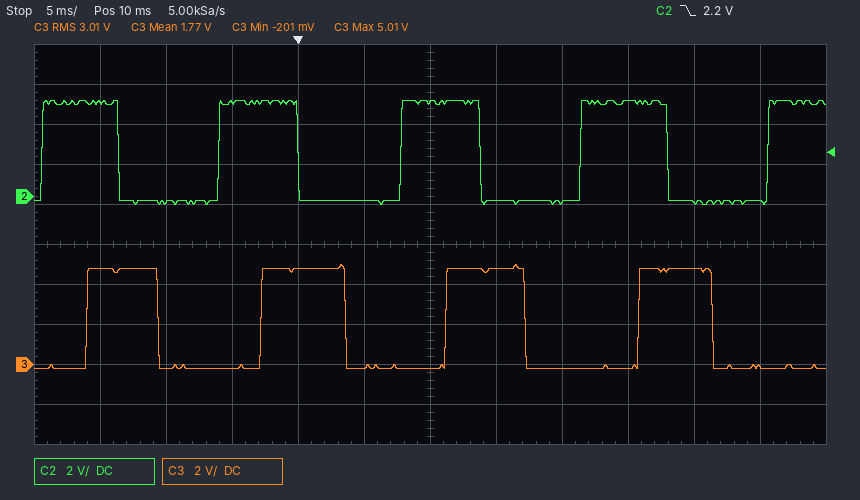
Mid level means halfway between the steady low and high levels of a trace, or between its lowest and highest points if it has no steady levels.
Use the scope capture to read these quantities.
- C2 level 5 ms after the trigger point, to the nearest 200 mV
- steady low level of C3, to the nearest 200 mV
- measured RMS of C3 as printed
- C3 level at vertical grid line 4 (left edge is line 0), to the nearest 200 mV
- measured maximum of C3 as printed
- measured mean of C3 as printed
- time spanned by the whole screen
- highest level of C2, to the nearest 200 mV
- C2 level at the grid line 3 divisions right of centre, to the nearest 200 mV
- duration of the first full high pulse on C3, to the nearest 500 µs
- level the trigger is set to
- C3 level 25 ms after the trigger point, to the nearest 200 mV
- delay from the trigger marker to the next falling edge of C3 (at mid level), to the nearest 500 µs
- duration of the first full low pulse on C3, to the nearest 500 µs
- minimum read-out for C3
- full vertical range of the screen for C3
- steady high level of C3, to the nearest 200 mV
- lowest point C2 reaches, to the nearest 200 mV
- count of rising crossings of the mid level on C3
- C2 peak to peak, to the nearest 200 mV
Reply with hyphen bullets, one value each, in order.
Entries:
- -200 mV
- -200 mV
- 3.01 V
- 4.8 V
- 5.01 V
- 1.77 V
- 60 ms
- 4.8 V
- 4.8 V
- 5.5 ms
- 2.2 V
- -200 mV
- 3.5 ms
- 8.0 ms
- -201 mV
- 20 V
- 4.8 V
- -400 mV
- 4
- 5.2 V
